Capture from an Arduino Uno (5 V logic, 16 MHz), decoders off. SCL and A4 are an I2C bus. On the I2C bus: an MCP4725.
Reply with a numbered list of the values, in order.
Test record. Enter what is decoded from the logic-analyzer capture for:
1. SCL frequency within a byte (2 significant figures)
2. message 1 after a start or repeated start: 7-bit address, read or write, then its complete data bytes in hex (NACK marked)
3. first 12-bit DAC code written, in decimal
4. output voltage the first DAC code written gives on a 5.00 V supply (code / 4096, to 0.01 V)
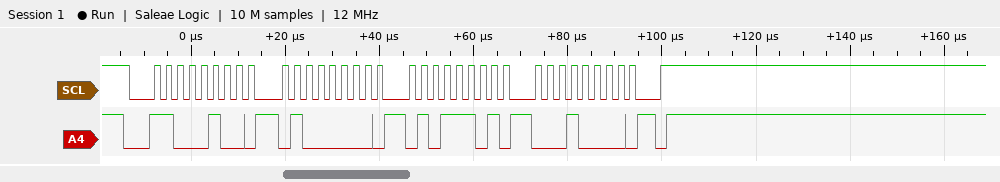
1. 400 kHz
2. 0x62 write: 40 5D 10
3. 1489
4. 1.82 V
